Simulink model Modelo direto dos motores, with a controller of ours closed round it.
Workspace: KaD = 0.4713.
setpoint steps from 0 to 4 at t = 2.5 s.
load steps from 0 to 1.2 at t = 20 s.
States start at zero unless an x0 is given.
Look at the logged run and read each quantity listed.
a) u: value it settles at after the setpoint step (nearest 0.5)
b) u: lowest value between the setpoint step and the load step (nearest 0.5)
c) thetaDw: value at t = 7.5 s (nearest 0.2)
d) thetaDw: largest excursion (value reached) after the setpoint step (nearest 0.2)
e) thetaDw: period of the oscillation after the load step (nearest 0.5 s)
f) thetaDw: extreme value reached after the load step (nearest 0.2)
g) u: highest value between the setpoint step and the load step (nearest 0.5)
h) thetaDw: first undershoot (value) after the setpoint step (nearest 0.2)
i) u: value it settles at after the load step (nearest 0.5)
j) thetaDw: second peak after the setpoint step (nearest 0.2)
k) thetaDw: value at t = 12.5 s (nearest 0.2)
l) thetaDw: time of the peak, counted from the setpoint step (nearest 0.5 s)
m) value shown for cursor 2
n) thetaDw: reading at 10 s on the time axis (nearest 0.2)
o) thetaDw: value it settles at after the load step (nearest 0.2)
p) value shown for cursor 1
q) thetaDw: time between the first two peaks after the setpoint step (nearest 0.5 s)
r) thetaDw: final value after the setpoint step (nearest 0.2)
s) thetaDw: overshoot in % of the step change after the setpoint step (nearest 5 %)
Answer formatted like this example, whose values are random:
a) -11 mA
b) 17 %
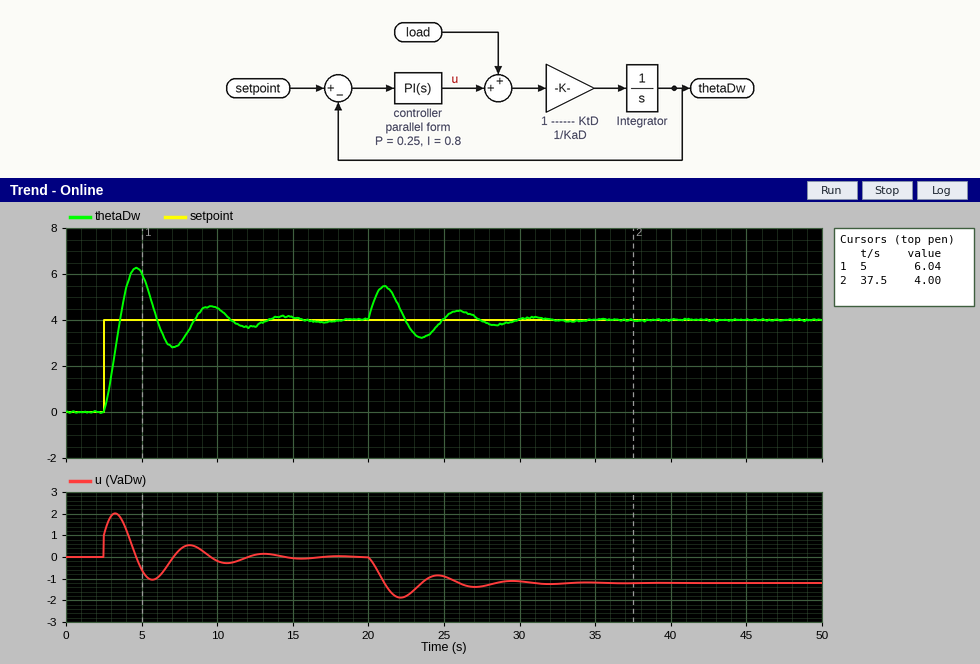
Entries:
a) 0.0
b) -1.0
c) 3.0
d) 6.2
e) 5.0 s
f) 5.4
g) 2.0
h) 2.8
i) -1.0
j) 4.6
k) 3.8
l) 2.0 s
m) 4.00
n) 4.6
o) 4.0
p) 6.04
q) 5.0 s
r) 4.0
s) 55 %
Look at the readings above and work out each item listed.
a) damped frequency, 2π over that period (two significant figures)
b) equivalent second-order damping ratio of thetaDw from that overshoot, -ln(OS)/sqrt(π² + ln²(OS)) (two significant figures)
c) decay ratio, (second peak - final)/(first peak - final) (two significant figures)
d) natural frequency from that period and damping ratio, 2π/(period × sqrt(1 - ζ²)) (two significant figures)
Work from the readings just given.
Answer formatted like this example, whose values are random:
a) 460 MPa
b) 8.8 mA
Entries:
a) 1.3 rad/s
b) 0.19
c) 0.27
d) 1.3 rad/s
